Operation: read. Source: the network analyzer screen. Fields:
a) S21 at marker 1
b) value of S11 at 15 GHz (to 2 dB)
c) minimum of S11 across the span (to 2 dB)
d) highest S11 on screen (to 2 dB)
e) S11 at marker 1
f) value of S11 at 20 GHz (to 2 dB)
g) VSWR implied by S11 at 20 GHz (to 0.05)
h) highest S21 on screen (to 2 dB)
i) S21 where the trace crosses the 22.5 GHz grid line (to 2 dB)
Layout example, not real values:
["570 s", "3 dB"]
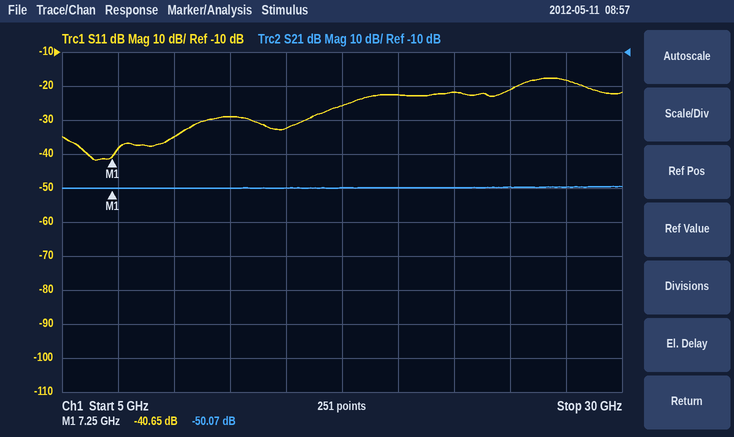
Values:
["-50.07 dB", "-32 dB", "-42 dB", "-18 dB", "-40.65 dB", "-22 dB", "1.15", "-50 dB", "-50 dB"]
